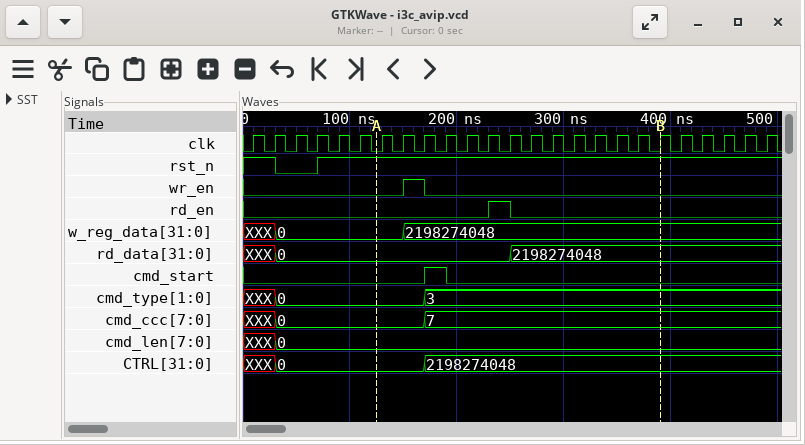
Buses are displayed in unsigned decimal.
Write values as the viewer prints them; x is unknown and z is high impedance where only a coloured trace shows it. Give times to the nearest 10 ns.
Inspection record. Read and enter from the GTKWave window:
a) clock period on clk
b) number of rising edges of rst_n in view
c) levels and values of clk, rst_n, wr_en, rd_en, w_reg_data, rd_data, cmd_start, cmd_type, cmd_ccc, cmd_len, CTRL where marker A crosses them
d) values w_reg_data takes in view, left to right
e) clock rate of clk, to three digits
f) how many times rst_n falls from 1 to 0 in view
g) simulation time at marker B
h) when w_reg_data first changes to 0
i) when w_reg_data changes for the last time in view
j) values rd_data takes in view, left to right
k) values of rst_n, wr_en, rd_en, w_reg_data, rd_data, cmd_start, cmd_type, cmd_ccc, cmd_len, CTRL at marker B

20 ns
1
clk=0, rst_n=1, wr_en=0, rd_en=0, w_reg_data=0, rd_data=0, cmd_start=0, cmd_type=0, cmd_ccc=0, cmd_len=0, CTRL=0
XXX, 0, 2198274048
50.0 MHz
1
390 ns
30 ns
150 ns
XXX, 0, 2198274048
rst_n=1, wr_en=0, rd_en=0, w_reg_data=2198274048, rd_data=2198274048, cmd_start=0, cmd_type=3, cmd_ccc=7, cmd_len=0, CTRL=2198274048
